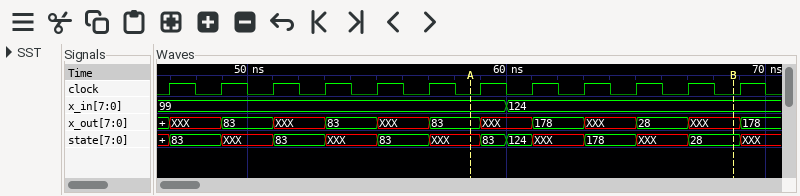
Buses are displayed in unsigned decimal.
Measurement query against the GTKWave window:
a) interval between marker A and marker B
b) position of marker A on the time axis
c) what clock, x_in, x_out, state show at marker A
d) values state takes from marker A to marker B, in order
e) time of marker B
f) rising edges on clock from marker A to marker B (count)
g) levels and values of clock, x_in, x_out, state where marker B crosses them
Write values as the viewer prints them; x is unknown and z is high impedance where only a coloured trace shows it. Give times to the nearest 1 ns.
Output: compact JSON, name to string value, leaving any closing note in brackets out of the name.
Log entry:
{"interval between marker A and marker B": "10 ns", "position of marker A on the time axis": "59 ns", "what clock, x_in, x_out, state show at marker A": "clock=0, x_in=99, x_out=83, state=XXX", "values state takes from marker A to marker B, in order": "XXX, 83, 124, XXX, 178, XXX, 28", "time of marker B": "69 ns", "rising edges on clock from marker A to marker B": "5", "levels and values of clock, x_in, x_out, state where marker B crosses them": "clock=0, x_in=124, x_out=XXX, state=28"}
